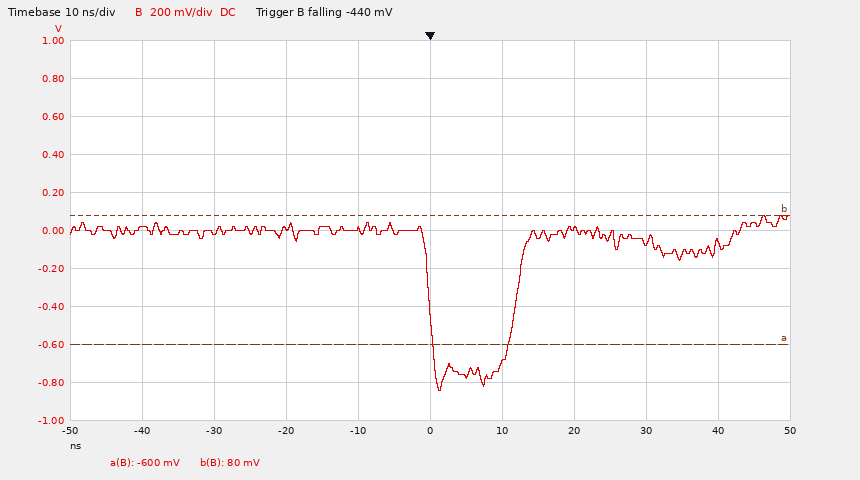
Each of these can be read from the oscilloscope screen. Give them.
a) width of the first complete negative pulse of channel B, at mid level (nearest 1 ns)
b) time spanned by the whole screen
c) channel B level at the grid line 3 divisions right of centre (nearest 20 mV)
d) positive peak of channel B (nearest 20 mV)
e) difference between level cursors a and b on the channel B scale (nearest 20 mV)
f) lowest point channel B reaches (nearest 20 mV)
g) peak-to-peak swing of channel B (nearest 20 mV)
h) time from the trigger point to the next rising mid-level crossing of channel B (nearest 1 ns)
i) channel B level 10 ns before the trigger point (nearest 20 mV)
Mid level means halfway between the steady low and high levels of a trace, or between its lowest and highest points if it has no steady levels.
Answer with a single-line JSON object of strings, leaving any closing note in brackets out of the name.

{"width of the first complete negative pulse of channel B, at mid level": "12 ns", "time spanned by the whole screen": "100 ns", "channel B level at the grid line 3 divisions right of centre": "-60 mV", "positive peak of channel B": "80 mV", "difference between level cursors a and b on the channel B scale": "680 mV", "lowest point channel B reaches": "-840 mV", "peak-to-peak swing of channel B": "920 mV", "time from the trigger point to the next rising mid-level crossing of channel B": "12 ns", "channel B level 10 ns before the trigger point": "0 mV"}
